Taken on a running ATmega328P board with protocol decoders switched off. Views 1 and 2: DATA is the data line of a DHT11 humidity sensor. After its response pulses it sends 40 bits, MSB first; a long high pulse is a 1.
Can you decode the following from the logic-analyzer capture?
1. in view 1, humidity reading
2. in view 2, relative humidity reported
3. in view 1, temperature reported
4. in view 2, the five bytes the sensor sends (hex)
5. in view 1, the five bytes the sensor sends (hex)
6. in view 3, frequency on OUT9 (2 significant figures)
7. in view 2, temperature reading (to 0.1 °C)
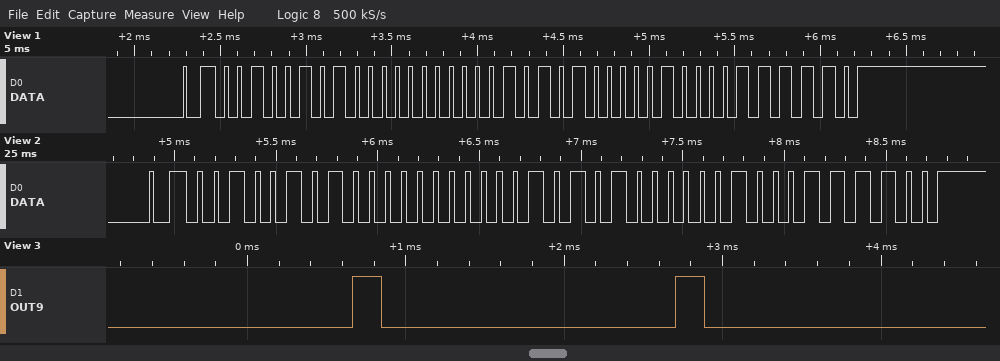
37 %
37 %
21.4 °C
25 00 15 02 3C
25 00 15 04 3E
490 Hz
21.2 °C
